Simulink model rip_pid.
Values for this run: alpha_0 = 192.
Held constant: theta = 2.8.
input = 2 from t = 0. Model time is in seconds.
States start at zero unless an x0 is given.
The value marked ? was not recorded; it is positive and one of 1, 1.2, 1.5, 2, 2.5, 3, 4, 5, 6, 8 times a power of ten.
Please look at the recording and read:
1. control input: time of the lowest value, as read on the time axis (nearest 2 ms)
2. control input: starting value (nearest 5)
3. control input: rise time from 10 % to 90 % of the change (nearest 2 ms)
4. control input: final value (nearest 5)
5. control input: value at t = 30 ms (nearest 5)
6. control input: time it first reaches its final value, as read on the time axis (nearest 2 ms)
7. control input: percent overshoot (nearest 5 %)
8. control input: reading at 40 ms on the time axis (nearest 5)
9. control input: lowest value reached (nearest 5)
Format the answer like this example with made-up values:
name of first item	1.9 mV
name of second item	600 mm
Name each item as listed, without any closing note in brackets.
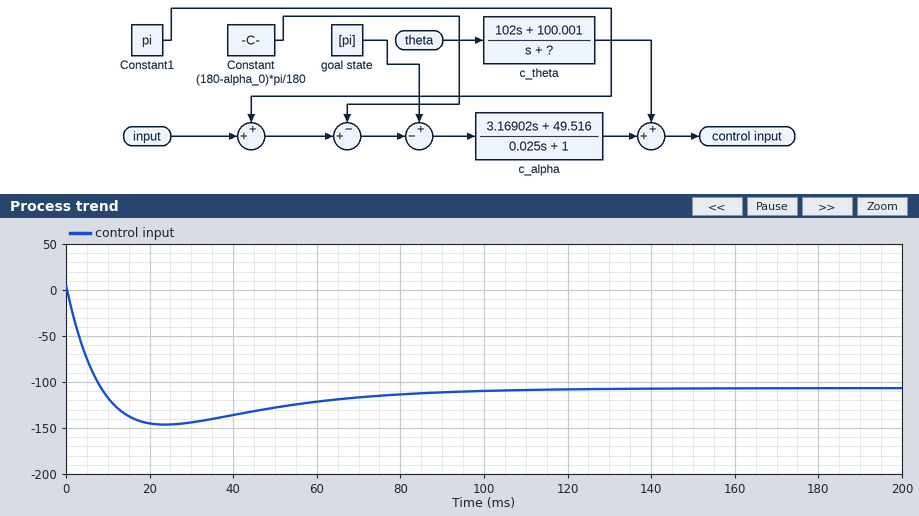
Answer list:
control input: time of the lowest value, as read on the time axis	24 ms
control input: starting value	5
control input: rise time from 10 % to 90 % of the change	6 ms
control input: final value	-105
control input: value at t = 30 ms	-145
control input: time it first reaches its final value, as read on the time axis	8 ms
control input: percent overshoot	35 %
control input: reading at 40 ms on the time axis	-135
control input: lowest value reached	-145
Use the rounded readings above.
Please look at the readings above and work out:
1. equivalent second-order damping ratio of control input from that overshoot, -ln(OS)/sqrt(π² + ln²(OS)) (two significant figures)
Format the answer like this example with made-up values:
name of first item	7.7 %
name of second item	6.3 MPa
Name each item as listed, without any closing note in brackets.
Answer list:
equivalent second-order damping ratio of control input from that overshoot, -ln(OS)/sqrt(π² + ln²(OS))	0.32
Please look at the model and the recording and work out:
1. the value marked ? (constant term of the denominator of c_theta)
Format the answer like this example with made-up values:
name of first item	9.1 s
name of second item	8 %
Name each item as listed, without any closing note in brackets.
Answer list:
the value marked ?	100
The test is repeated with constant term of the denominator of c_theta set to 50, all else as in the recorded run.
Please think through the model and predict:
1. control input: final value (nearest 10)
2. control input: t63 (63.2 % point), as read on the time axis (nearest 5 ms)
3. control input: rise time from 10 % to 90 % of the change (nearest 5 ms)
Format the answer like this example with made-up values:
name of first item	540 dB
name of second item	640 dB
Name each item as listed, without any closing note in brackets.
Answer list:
control input: final value	-100
control input: t63 (63.2 % point), as read on the time axis	15 ms
control input: rise time from 10 % to 90 % of the change	30 ms
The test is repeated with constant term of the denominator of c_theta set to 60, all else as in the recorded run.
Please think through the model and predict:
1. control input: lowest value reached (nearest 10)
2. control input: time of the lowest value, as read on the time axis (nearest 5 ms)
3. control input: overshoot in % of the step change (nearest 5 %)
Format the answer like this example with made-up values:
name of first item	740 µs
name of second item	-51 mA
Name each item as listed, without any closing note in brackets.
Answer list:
control input: lowest value reached	-110
control input: time of the lowest value, as read on the time axis	45 ms
control input: overshoot in % of the step change	10 %
